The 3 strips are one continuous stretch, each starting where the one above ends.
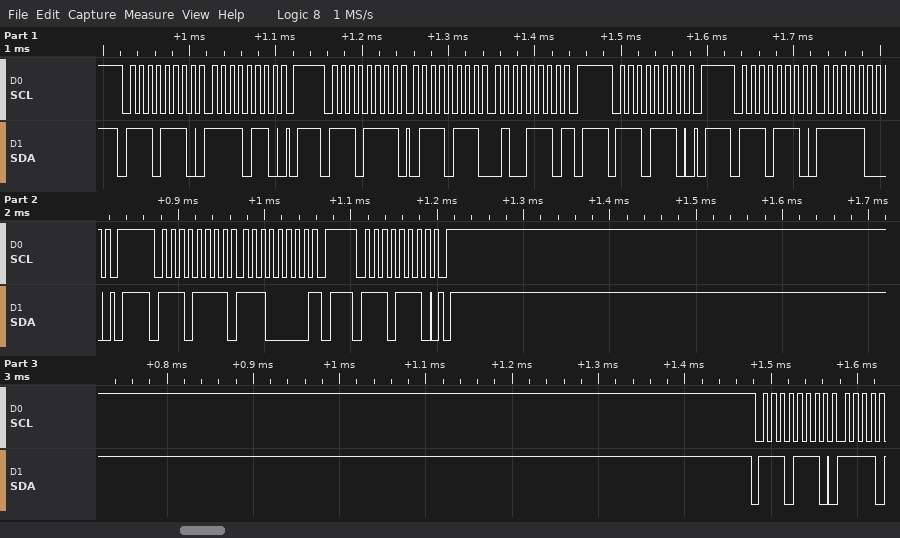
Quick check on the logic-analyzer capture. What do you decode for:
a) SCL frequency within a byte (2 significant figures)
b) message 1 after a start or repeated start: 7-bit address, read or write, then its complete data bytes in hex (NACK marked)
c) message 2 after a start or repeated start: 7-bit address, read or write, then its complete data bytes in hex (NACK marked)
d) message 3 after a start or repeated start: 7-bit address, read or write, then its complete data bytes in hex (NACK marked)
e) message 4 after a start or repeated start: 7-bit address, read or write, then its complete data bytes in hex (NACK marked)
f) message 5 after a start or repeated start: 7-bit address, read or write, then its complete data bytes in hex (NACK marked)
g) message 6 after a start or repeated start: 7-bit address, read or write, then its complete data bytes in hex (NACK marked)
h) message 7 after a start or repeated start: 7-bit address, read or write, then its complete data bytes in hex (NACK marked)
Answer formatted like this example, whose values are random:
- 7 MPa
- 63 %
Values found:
- 100 kHz
- 0x77 write: F6
- 0x77 read: 77 4E NACK
- 0x77 write
- 0x77 write: F8
- 0x77 read: E0 NACK
- 0x77 write
- 0x77 write
